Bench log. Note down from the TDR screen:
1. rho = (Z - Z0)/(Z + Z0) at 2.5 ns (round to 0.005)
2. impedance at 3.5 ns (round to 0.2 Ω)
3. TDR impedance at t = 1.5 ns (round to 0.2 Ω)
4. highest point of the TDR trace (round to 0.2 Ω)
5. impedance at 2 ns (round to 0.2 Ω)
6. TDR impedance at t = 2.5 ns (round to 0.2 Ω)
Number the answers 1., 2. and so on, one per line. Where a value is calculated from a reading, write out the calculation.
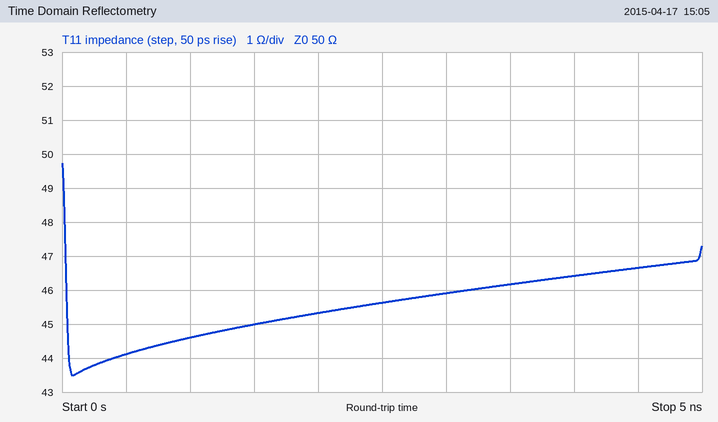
1. (45.6 − 50)/(45.6 + 50) ≈ -0.0460, so -0.045 to the nearest 0.005
2. 46.2 Ω
3. 45.0 Ω
4. 49.8 Ω
5. 45.4 Ω
6. 45.6 Ω
